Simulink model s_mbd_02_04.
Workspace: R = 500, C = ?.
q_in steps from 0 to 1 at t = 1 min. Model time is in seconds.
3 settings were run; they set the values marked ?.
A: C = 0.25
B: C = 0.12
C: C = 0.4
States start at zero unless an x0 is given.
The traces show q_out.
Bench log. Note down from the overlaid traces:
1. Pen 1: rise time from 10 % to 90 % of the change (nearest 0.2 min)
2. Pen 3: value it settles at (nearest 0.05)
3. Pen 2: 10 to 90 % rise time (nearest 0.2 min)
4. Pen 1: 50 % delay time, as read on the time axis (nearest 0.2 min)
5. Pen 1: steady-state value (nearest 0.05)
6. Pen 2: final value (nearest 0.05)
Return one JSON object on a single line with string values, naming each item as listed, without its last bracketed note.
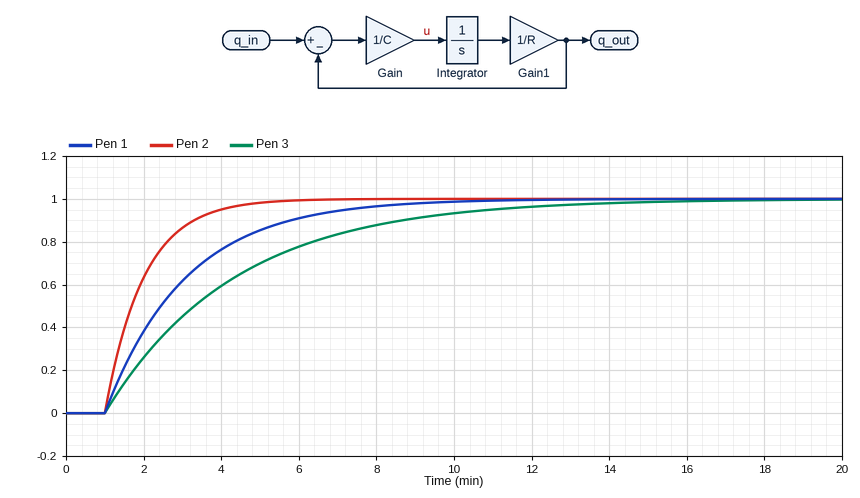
{"Pen 1: rise time from 10 % to 90 % of the change": "4.6 min", "Pen 3: value it settles at": "1.00", "Pen 2: 10 to 90 % rise time": "2.2 min", "Pen 1: 50 % delay time, as read on the time axis": "2.4 min", "Pen 1: steady-state value": "1.00", "Pen 2: final value": "1.00"}
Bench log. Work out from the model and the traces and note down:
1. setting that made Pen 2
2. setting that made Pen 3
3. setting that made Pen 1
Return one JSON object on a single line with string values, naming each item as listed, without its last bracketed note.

{"setting that made Pen 2": "B", "setting that made Pen 3": "C", "setting that made Pen 1": "A"}
